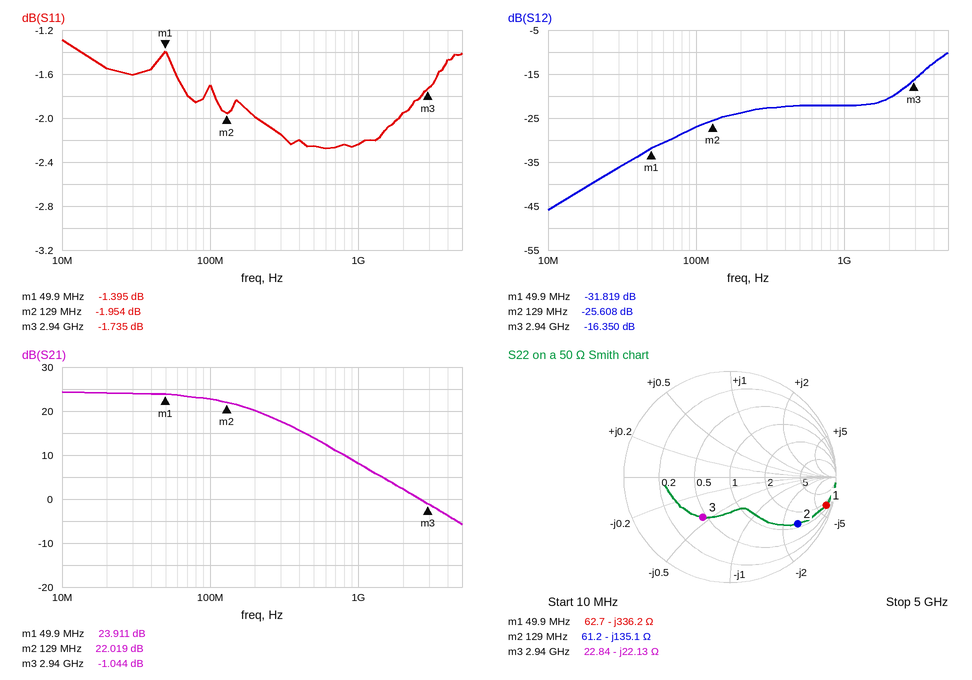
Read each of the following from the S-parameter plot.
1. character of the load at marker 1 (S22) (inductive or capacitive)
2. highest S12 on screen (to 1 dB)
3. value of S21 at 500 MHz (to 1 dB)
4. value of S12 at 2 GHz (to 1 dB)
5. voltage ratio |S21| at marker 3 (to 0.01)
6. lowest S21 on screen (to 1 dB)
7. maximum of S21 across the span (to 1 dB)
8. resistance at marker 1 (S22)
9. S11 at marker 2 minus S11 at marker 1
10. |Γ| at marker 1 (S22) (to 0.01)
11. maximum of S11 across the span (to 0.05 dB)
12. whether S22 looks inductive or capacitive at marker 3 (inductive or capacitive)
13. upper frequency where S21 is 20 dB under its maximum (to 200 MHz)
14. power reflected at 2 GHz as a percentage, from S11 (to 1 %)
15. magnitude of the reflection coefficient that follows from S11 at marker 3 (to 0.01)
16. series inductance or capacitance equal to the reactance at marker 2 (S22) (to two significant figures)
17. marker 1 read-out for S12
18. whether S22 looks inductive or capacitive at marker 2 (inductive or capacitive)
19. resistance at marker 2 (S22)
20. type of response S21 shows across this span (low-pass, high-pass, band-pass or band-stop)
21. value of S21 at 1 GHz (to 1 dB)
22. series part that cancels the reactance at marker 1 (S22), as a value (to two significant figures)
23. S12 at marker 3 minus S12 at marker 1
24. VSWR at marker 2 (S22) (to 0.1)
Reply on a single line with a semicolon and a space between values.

capacitive; -10 dB; 14 dB; -20 dB; 0.89; -6 dB; 24 dB; 62.7 Ω; -0.559 dB; 0.95; -1.30 dB; capacitive; 1.6 GHz; 64 %; 0.82; 9.1 pF; -31.819 dB; capacitive; 61.2 Ω; low-pass; 8 dB; 1.1 µH; 15.469 dB; 7.9
